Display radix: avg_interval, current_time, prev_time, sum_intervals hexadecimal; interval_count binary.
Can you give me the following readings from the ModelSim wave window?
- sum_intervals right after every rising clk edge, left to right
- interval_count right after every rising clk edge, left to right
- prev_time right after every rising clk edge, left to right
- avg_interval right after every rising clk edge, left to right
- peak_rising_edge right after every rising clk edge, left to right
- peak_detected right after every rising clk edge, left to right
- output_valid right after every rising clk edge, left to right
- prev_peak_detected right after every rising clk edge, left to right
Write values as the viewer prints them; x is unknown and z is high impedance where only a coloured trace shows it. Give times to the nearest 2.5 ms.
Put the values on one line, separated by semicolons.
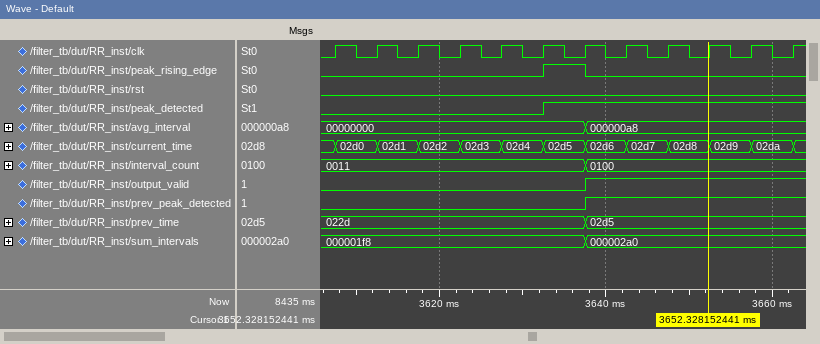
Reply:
000001f8, 000001f8, 000001f8, 000001f8, 000001f8, 000001f8, 000002a0, 000002a0, 000002a0, 000002a0, 000002a0, 000002a0; 0011, 0011, 0011, 0011, 0011, 0011, 0100, 0100, 0100, 0100, 0100, 0100; 022d, 022d, 022d, 022d, 022d, 022d, 02d5, 02d5, 02d5, 02d5, 02d5, 02d5; 00000000, 00000000, 00000000, 00000000, 00000000, 00000000, 000000a8, 000000a8, 000000a8, 000000a8, 000000a8, 000000a8; 0 0 0 0 0 1 0 0 0 0 0 0; 0 0 0 0 0 1 1 1 1 1 1 1; 0 0 0 0 0 0 1 1 1 1 1 1; 0 0 0 0 0 0 1 1 1 1 1 1
